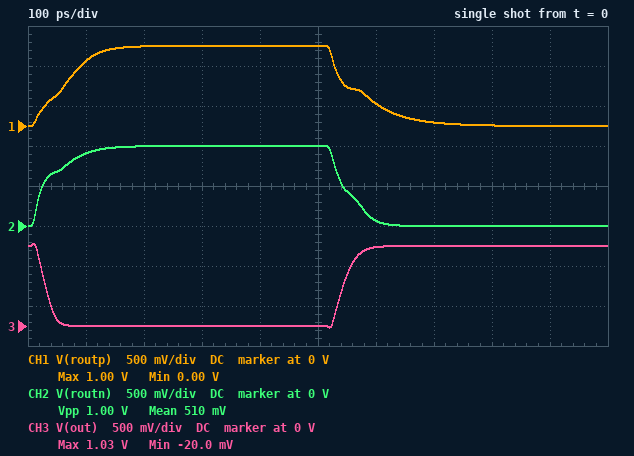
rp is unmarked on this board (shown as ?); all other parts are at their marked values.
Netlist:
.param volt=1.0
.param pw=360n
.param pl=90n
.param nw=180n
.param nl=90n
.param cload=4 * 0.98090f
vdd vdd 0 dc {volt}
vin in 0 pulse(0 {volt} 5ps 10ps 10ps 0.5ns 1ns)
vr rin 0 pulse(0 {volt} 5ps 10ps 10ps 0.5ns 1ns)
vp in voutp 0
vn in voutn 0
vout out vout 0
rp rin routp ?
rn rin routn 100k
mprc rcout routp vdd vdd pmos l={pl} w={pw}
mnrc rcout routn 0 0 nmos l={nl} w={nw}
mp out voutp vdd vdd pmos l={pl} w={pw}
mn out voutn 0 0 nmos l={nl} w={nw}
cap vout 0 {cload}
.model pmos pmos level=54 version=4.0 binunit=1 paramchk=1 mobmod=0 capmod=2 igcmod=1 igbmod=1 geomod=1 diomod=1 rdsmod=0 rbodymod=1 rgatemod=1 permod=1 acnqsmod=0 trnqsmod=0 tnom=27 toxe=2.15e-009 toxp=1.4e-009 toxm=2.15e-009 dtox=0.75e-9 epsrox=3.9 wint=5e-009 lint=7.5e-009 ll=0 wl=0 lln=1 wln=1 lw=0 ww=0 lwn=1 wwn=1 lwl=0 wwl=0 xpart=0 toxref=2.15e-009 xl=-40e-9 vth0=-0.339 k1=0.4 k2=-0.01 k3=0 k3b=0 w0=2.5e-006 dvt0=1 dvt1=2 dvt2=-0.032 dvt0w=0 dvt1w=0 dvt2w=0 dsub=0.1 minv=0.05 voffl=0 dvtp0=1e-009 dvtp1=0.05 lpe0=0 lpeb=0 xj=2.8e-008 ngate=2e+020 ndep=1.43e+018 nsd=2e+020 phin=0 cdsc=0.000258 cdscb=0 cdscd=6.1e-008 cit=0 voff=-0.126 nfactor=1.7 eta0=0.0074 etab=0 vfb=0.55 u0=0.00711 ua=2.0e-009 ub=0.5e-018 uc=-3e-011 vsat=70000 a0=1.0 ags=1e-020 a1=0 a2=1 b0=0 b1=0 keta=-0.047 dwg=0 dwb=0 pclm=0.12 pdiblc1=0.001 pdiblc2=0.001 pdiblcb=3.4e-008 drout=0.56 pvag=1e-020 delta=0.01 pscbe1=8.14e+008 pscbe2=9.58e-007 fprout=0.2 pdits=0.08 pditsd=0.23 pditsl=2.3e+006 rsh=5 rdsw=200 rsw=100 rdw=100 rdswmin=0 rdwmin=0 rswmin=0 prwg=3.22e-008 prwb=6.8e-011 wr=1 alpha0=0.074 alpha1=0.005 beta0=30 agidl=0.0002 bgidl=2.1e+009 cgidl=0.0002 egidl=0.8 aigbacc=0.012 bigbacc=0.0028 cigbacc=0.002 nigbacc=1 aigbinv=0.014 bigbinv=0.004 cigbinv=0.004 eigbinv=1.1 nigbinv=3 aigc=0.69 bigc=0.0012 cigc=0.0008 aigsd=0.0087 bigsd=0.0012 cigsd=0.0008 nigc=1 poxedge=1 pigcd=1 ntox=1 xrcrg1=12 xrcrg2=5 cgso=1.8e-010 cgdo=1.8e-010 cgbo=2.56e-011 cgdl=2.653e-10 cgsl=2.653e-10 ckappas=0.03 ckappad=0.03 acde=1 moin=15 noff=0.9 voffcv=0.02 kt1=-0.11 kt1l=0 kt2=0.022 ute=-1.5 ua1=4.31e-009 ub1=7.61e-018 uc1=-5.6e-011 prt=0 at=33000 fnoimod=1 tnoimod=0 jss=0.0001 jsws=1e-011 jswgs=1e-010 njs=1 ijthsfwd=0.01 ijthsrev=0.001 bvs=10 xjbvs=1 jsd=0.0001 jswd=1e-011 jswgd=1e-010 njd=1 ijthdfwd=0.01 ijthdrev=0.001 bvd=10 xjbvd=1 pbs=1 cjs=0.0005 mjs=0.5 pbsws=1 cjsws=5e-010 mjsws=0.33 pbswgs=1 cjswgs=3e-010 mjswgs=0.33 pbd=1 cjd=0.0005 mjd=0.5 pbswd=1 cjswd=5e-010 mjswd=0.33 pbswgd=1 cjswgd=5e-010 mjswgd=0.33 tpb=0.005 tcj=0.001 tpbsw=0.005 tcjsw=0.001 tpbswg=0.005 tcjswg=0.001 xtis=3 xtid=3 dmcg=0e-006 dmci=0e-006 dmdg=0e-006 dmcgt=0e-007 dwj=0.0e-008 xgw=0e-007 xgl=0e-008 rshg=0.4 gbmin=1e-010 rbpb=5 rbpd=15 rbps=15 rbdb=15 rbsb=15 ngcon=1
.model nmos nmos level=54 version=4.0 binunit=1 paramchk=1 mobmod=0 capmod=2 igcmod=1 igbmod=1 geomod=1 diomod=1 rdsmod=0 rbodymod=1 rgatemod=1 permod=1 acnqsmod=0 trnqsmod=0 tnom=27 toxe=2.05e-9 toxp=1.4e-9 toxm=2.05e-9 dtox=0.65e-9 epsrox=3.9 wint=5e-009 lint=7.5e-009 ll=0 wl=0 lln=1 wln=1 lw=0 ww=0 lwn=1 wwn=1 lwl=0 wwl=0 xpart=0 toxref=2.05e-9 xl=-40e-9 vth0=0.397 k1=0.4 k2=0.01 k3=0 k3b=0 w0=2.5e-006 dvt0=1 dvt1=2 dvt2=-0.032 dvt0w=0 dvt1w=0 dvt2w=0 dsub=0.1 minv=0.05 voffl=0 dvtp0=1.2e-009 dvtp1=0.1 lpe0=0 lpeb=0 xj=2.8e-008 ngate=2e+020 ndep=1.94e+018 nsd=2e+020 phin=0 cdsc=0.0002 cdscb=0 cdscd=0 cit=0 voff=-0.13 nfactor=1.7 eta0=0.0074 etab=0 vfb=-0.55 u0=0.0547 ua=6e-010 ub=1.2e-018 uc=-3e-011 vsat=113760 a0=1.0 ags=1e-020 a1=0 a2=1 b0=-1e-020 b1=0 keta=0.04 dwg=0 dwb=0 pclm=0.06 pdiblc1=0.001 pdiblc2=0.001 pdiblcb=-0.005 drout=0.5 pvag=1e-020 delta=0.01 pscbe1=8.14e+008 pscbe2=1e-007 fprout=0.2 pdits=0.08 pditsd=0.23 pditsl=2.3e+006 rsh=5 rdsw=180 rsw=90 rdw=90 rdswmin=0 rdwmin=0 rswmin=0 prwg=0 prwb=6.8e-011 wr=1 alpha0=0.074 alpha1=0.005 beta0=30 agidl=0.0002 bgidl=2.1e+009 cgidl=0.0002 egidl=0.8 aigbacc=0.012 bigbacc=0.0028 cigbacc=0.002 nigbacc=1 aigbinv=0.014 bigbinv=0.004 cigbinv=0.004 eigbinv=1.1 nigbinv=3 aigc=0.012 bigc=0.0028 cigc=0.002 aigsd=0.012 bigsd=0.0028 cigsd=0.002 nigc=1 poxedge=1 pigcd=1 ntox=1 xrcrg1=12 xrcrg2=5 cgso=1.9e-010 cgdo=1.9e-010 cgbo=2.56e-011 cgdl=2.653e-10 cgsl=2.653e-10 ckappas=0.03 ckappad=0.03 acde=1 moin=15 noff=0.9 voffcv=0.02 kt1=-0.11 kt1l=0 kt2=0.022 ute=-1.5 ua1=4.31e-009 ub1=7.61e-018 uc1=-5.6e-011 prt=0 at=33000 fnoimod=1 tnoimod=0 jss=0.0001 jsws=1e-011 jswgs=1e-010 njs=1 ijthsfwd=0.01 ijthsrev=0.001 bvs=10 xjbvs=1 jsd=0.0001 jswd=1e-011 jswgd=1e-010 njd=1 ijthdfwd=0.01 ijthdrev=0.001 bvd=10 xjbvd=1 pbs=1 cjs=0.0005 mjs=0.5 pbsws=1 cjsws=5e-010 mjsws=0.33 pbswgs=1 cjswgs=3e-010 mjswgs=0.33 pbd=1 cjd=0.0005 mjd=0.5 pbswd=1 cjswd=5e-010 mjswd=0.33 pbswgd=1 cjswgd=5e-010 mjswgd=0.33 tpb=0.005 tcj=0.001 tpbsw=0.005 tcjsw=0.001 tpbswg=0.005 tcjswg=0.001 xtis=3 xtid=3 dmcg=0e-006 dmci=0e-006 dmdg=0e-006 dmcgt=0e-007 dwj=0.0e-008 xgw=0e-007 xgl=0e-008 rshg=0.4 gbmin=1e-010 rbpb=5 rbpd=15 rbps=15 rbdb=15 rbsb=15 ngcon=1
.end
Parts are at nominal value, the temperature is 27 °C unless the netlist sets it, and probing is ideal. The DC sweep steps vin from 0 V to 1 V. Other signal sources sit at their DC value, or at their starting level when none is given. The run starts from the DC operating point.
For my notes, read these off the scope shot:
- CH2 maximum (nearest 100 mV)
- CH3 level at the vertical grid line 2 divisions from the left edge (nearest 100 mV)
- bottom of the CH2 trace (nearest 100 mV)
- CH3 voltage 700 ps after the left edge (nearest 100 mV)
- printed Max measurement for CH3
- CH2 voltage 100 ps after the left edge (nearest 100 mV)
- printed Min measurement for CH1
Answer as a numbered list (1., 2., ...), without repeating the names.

1. 1.0 V
2. 0 V
3. 0 V
4. 1.0 V
5. 1.03 V
6. 900 mV
7. 0.00 V
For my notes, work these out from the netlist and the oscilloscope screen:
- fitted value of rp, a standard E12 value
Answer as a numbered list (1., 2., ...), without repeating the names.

1. 82 kΩ
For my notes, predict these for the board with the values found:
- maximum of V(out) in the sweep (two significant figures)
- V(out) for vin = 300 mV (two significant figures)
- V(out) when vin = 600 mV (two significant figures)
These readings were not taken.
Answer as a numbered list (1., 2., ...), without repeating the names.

1. 1.0 V
2. 980 mV
3. 40 mV
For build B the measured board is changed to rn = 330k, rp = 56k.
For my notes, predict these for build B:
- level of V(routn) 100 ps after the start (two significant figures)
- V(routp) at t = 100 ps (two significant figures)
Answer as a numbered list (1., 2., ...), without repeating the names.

1. 510 mV
2. 900 mV
